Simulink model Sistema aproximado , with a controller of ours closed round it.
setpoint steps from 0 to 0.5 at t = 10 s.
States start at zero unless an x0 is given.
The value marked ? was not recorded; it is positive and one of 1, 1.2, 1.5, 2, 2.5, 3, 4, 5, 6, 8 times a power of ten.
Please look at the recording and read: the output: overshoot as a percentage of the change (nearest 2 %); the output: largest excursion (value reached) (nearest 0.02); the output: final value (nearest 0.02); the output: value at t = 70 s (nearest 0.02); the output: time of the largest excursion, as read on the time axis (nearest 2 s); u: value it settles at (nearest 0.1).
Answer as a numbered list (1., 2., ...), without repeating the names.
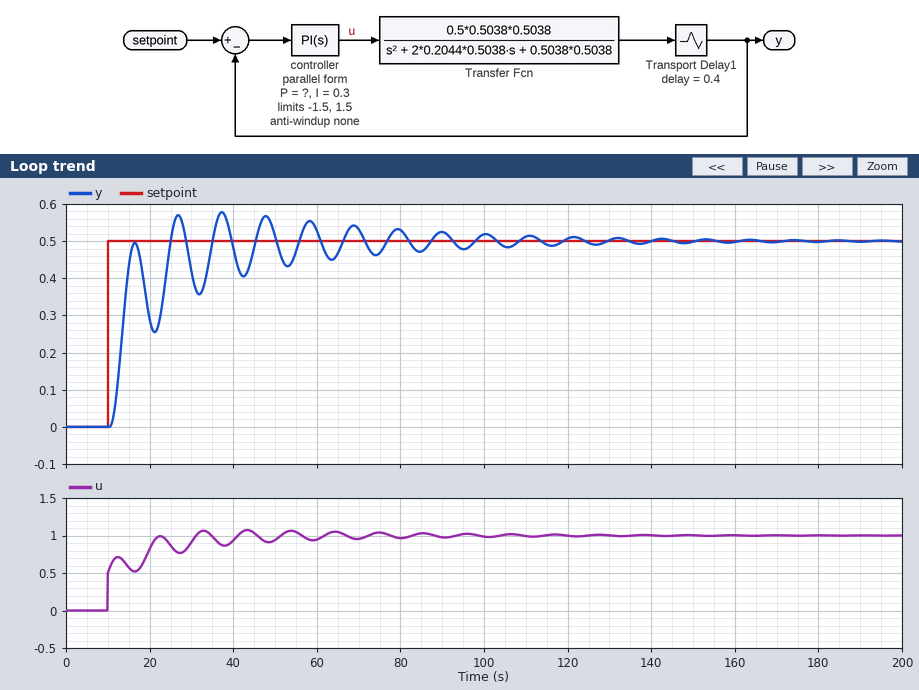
1. 16 %
2. 0.58
3. 0.50
4. 0.54
5. 38 s
6. 1.0
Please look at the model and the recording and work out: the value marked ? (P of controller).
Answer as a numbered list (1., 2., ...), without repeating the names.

1. 1
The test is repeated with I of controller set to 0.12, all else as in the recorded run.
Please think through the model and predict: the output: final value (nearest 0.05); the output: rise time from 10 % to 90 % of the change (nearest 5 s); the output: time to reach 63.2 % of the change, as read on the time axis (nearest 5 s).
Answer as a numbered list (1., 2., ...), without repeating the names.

1. 0.50
2. 45 s
3. 15 s
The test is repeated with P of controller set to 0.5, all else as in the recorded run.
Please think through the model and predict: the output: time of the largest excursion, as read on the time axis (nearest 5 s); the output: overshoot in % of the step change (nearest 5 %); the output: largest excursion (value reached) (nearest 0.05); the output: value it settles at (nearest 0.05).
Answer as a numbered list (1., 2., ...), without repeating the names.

1. 40 s
2. 10 %
3. 0.55
4. 0.50
